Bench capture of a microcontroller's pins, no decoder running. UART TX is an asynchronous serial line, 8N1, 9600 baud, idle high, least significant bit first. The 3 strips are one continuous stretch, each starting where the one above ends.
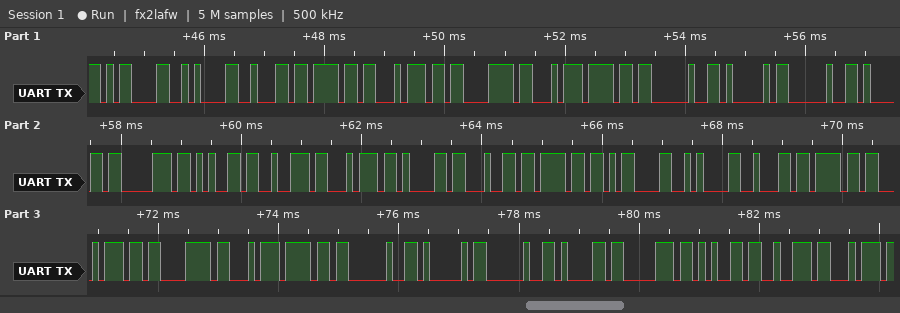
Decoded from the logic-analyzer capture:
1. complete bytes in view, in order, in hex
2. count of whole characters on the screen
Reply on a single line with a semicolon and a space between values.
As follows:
0x0D 0x0A 0x62 0x6F 0x74 0xC3 0xA3 0x6F 0x20 0x41 0x20 0x61 0x70 0x65 0x72 0x74 0x61 0x64 0x6F 0x0D 0x0A 0x62 0x6F 0x74 0xC3 0xA3 0x6F 0x20 0x41 0x20 0x61 0x70 0x65 0x72 0x74; 35
